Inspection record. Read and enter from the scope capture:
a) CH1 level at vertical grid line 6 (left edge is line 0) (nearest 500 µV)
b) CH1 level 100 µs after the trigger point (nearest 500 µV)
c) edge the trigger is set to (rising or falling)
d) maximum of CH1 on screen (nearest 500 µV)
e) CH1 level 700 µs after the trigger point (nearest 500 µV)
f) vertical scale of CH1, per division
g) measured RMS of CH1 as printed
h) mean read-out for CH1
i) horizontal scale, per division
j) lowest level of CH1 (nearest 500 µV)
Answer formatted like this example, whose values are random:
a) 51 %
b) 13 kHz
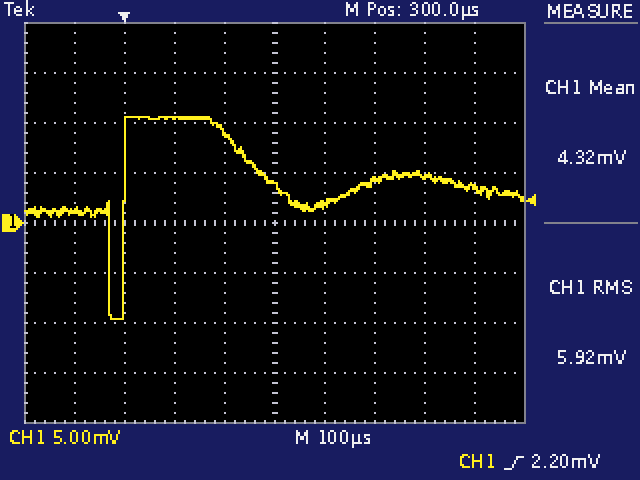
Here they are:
a) 2.0 mV
b) 10.5 mV
c) rising
d) 10.5 mV
e) 3.5 mV
f) 5 mV
g) 5.92 mV
h) 4.32 mV
i) 100 µs
j) -9.5 mV
